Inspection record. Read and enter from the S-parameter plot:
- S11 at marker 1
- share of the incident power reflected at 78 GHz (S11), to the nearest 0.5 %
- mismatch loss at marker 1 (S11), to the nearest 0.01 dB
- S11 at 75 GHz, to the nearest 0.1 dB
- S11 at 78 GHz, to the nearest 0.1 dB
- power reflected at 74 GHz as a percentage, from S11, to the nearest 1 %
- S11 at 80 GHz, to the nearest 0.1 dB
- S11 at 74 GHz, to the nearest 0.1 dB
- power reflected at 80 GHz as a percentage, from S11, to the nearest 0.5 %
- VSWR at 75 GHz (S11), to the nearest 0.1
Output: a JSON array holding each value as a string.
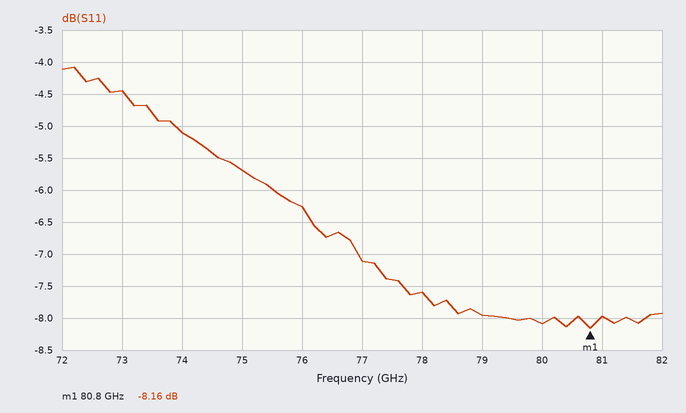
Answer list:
["-8.16 dB", "17.5 %", "0.72 dB", "-5.7 dB", "-7.6 dB", "31 %", "-8.1 dB", "-5.1 dB", "15.5 %", "3.2"]
